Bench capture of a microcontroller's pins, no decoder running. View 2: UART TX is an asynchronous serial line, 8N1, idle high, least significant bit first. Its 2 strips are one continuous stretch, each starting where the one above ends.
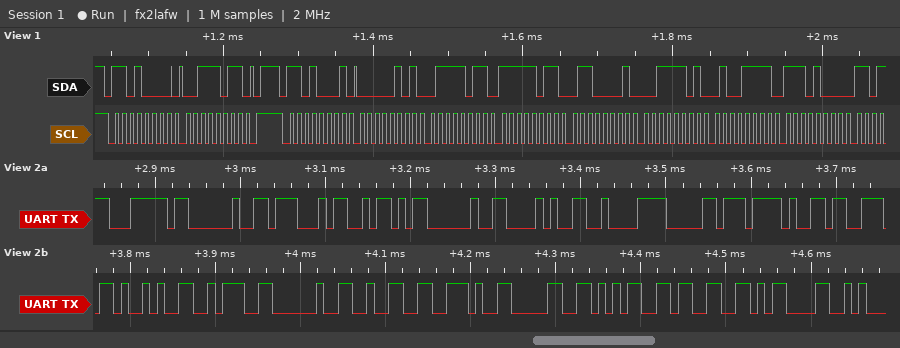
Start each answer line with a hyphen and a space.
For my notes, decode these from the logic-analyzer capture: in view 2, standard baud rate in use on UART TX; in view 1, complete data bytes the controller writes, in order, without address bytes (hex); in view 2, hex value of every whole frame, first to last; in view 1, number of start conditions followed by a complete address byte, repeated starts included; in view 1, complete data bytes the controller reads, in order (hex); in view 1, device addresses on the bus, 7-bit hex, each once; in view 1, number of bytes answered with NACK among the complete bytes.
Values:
- 115200 baud
- 3B
- 7C 20 47 5A 20 28 C2 B0 2F 73 29 3A 20 32 2E 30 35 33 0D
- 2
- 05 7B FB 61 3D 4F E8
- 0x68
- 0
